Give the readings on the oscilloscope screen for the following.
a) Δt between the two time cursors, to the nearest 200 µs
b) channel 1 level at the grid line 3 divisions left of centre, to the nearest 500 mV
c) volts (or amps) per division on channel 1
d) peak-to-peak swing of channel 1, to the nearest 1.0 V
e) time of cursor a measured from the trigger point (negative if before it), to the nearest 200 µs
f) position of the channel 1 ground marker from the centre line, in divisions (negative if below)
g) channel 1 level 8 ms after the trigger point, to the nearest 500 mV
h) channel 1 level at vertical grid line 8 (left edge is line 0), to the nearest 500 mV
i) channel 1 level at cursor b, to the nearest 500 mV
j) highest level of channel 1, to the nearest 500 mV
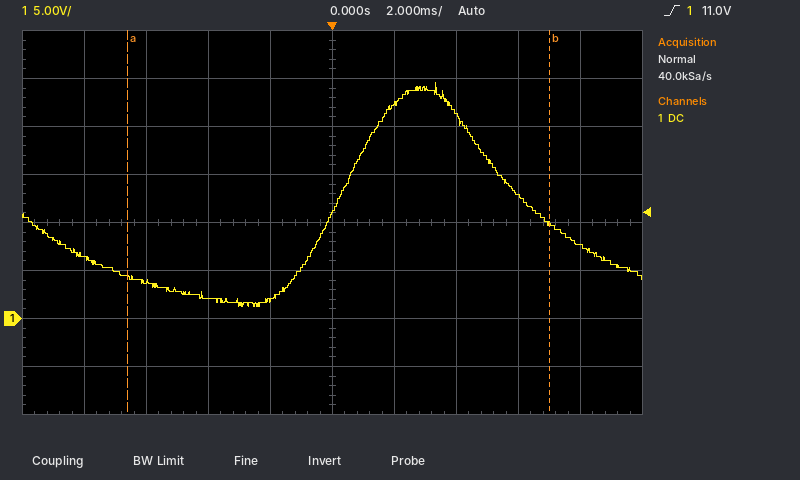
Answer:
13.6 ms
4.0 V
5 V
23.0 V
-6.6 ms
-2.0 div
7.5 V
13.0 V
10.0 V
24.5 V
